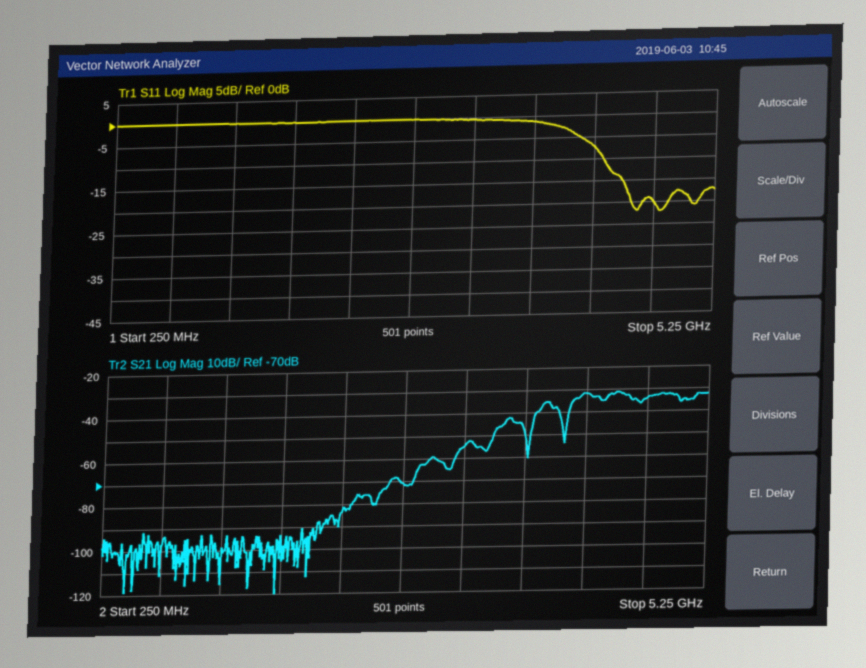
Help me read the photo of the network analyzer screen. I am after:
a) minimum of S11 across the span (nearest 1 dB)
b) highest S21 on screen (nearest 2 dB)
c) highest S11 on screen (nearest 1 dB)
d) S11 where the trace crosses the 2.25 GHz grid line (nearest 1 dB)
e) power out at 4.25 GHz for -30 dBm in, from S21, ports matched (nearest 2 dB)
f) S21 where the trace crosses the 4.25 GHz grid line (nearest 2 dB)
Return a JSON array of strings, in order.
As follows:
["-22 dB", "-32 dB", "0 dB", "0 dB", "-62 dBm", "-32 dB"]
